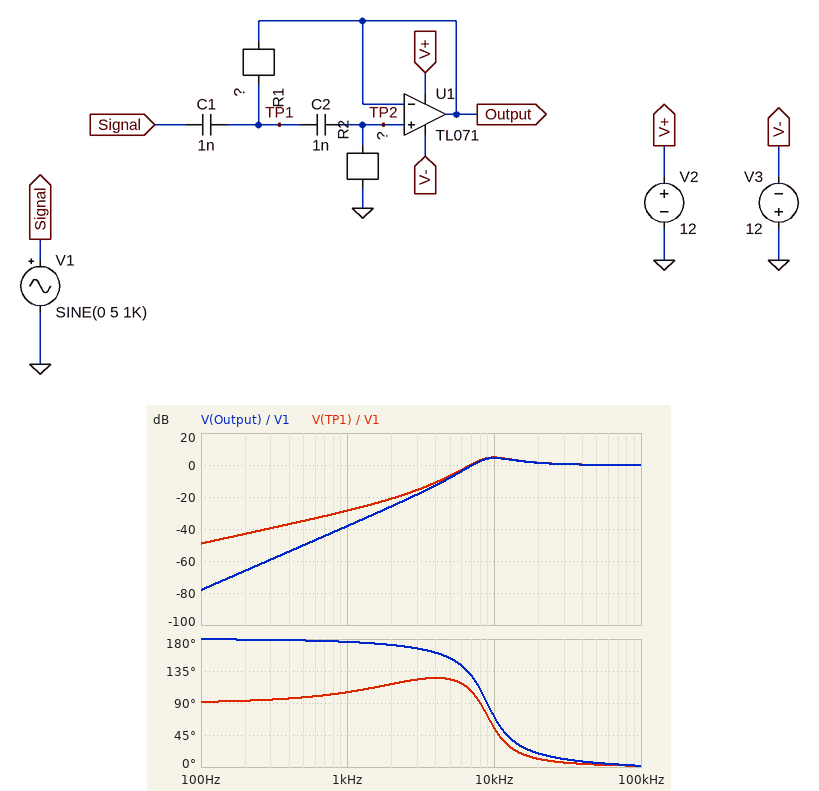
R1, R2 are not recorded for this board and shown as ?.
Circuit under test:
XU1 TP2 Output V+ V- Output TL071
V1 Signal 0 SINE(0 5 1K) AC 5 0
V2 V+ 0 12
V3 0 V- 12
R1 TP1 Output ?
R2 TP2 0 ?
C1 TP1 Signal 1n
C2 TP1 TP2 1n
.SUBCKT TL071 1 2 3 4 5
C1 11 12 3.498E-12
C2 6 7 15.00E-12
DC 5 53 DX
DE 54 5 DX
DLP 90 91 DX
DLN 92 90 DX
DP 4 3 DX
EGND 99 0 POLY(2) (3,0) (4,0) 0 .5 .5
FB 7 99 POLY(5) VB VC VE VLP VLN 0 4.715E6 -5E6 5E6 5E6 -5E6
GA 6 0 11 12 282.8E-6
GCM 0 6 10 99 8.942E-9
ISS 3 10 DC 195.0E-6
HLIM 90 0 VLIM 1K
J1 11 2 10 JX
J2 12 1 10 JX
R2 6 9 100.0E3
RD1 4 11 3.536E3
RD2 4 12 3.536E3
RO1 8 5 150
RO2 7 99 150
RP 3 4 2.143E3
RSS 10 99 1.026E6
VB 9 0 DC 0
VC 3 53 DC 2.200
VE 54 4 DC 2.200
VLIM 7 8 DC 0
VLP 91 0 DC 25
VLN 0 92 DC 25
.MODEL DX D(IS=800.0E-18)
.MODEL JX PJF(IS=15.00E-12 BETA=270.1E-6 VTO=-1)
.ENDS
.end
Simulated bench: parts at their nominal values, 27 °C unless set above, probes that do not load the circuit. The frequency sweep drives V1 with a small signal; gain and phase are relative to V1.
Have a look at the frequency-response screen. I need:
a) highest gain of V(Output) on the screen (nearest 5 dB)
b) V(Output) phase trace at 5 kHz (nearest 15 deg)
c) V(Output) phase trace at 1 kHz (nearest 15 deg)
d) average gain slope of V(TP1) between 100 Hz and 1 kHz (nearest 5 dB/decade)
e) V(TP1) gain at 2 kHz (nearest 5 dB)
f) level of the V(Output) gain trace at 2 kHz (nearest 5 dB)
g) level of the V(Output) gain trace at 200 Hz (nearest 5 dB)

5 dB
150 deg
180 deg
20 dB/decade
-20 dB
-25 dB
-65 dB
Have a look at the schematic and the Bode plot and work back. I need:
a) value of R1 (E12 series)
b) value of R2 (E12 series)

5.6 kΩ
56 kΩ
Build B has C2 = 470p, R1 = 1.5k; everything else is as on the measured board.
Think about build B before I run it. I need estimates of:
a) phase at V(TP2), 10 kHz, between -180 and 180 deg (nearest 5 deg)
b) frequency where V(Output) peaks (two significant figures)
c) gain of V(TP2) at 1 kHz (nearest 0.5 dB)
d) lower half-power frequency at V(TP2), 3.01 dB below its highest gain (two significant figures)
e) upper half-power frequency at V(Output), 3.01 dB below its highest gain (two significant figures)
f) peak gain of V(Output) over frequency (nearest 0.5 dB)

170 deg
26 kHz
-56.0 dB
22 kHz
32 kHz
9.0 dB
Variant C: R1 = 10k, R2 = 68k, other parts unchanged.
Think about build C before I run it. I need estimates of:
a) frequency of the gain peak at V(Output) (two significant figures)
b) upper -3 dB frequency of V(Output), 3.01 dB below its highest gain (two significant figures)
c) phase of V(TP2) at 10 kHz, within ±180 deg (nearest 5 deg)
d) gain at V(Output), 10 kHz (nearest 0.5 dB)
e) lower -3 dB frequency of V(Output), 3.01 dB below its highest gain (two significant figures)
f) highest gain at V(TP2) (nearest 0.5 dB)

7.2 kHz
1.3 MHz
35 deg
2.0 dB
5.1 kHz
3.0 dB
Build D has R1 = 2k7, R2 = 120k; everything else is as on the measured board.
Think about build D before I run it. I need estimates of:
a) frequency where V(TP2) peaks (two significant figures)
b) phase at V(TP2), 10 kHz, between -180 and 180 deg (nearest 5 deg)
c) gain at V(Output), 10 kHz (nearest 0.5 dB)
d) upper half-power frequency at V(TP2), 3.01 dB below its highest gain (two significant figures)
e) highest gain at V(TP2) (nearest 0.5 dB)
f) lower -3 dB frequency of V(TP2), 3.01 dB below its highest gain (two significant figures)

9.0 kHz
50 deg
9.0 dB
11 kHz
10.5 dB
7.8 kHz
